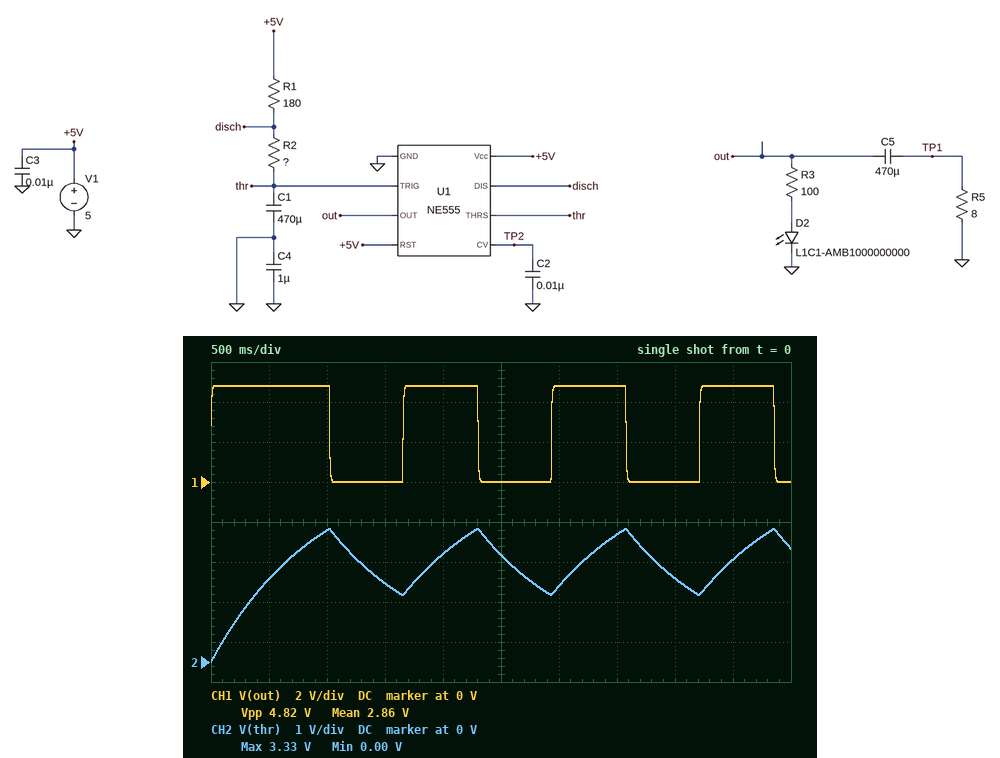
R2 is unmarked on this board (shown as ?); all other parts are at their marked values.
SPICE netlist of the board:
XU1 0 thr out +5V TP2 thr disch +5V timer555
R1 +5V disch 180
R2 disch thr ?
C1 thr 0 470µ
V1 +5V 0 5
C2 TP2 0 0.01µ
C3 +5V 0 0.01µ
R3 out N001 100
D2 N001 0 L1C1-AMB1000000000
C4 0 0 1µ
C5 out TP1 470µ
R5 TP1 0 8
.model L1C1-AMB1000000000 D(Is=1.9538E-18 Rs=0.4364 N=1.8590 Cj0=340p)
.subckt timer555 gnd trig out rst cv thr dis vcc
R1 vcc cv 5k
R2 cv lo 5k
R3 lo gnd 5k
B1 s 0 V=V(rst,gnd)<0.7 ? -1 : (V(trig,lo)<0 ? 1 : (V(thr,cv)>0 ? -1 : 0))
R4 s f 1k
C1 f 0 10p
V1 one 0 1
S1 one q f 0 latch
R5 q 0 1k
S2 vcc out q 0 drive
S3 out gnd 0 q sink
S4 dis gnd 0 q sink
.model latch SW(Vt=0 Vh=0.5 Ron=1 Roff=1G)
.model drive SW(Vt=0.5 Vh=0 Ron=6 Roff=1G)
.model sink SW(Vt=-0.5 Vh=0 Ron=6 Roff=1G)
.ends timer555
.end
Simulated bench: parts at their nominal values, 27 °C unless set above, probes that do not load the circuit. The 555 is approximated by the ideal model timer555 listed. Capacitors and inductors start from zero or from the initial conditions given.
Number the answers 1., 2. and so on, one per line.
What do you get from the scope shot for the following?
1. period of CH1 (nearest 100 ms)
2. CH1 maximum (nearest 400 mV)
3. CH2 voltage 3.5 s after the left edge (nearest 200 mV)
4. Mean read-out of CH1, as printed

1. 1.3 s
2. 4.8 V
3. 3.2 V
4. 2.86 V
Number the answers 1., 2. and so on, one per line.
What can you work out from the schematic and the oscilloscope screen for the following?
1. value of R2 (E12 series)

1. 1.8 kΩ
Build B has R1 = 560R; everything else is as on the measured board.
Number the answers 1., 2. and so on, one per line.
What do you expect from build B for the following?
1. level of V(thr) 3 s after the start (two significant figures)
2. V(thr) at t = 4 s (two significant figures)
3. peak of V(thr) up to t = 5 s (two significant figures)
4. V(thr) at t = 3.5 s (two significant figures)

1. 2.1 V
2. 3.2 V
3. 3.3 V
4. 2.5 V
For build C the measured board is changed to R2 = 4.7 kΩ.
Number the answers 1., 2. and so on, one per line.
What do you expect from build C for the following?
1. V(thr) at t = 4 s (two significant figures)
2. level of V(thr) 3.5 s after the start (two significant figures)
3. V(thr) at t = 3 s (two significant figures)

1. 1.8 V
2. 2.2 V
3. 2.7 V
